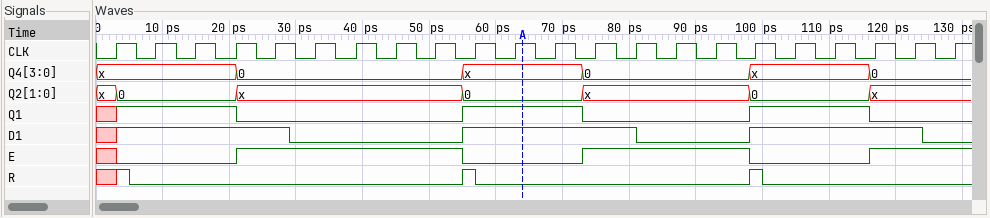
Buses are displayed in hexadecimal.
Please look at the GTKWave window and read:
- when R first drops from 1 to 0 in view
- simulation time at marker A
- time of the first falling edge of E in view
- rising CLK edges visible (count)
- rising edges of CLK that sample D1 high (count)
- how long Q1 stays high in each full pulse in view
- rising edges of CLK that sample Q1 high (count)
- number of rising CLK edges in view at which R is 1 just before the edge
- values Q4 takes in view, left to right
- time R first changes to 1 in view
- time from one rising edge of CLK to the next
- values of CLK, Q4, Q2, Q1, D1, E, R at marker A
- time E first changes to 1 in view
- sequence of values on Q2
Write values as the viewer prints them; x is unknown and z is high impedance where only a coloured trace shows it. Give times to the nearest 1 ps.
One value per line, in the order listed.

5 ps
64 ps
55 ps
22
14
18 ps, 18 ps
9
2
x, 0, x, 0, x, 0
3 ps
6 ps
CLK=1, Q4=x, Q2=0, Q1=1, D1=1, E=0, R=0
21 ps
x, 0, x, 0, x, 0, x
